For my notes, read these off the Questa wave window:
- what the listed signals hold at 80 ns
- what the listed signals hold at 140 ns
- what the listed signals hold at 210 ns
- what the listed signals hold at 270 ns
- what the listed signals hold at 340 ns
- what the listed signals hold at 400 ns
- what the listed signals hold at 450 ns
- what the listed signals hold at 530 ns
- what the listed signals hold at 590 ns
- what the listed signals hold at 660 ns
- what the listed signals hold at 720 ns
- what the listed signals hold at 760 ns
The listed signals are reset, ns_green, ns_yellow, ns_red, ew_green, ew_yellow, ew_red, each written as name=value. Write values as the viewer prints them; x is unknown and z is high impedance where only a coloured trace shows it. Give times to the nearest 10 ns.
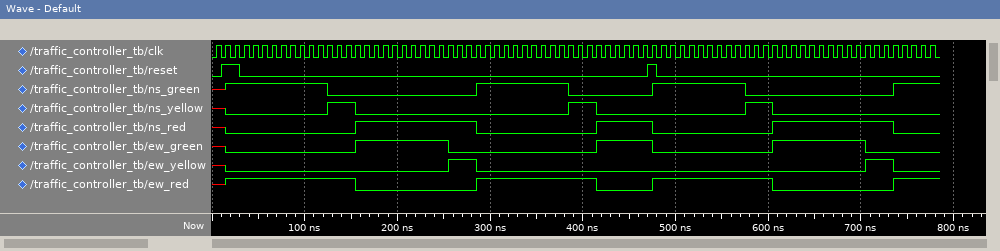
reset=0, ns_green=1, ns_yellow=0, ns_red=0, ew_green=0, ew_yellow=0, ew_red=1
reset=0, ns_green=0, ns_yellow=1, ns_red=0, ew_green=0, ew_yellow=0, ew_red=1
reset=0, ns_green=0, ns_yellow=0, ns_red=1, ew_green=1, ew_yellow=0, ew_red=0
reset=0, ns_green=0, ns_yellow=0, ns_red=1, ew_green=0, ew_yellow=1, ew_red=0
reset=0, ns_green=1, ns_yellow=0, ns_red=0, ew_green=0, ew_yellow=0, ew_red=1
reset=0, ns_green=0, ns_yellow=1, ns_red=0, ew_green=0, ew_yellow=0, ew_red=1
reset=0, ns_green=0, ns_yellow=0, ns_red=1, ew_green=1, ew_yellow=0, ew_red=0
reset=0, ns_green=1, ns_yellow=0, ns_red=0, ew_green=0, ew_yellow=0, ew_red=1
reset=0, ns_green=0, ns_yellow=1, ns_red=0, ew_green=0, ew_yellow=0, ew_red=1
reset=0, ns_green=0, ns_yellow=0, ns_red=1, ew_green=1, ew_yellow=0, ew_red=0
reset=0, ns_green=0, ns_yellow=0, ns_red=1, ew_green=0, ew_yellow=1, ew_red=0
reset=0, ns_green=1, ns_yellow=0, ns_red=0, ew_green=0, ew_yellow=0, ew_red=1
